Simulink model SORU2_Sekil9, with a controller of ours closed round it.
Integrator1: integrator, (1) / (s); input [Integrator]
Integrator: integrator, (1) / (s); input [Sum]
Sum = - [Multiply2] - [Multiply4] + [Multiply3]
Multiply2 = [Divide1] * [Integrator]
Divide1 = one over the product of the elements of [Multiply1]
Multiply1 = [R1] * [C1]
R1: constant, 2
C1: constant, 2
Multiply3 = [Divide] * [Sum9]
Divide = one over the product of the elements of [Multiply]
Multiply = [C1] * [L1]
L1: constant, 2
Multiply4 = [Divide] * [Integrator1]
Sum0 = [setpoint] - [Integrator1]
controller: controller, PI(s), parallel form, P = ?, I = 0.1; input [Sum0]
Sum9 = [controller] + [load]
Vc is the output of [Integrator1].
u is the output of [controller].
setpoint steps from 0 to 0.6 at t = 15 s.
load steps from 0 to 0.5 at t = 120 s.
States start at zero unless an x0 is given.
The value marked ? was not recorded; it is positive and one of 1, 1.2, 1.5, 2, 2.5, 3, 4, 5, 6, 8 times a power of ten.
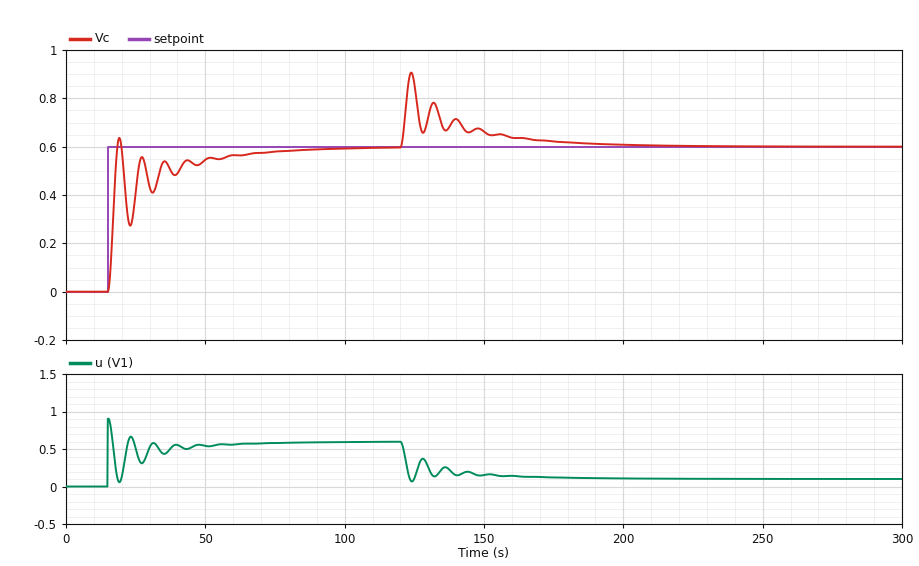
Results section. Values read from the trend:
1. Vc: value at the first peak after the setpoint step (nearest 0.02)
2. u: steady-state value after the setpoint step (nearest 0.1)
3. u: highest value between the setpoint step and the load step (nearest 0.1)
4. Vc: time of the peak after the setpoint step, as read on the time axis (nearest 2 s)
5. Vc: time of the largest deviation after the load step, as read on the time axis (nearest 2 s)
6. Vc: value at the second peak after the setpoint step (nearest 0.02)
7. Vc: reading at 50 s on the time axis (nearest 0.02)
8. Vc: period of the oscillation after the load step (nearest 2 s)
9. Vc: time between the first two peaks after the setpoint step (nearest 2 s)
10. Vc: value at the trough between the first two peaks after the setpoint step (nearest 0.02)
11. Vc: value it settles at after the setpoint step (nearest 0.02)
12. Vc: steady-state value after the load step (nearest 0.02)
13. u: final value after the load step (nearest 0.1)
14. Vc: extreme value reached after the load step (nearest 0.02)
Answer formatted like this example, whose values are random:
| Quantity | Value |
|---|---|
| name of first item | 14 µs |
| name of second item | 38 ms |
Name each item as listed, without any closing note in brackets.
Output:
| Quantity | Value |
|---|---|
| Vc: value at the first peak after the setpoint step | 0.64 |
| u: steady-state value after the setpoint step | 0.6 |
| u: highest value between the setpoint step and the load step | 0.9 |
| Vc: time of the peak after the setpoint step, as read on the time axis | 20 s |
| Vc: time of the largest deviation after the load step, as read on the time axis | 124 s |
| Vc: value at the second peak after the setpoint step | 0.56 |
| Vc: reading at 50 s on the time axis | 0.54 |
| Vc: period of the oscillation after the load step | 8 s |
| Vc: time between the first two peaks after the setpoint step | 8 s |
| Vc: value at the trough between the first two peaks after the setpoint step | 0.28 |
| Vc: value it settles at after the setpoint step | 0.60 |
| Vc: steady-state value after the load step | 0.60 |
| u: final value after the load step | 0.1 |
| Vc: extreme value reached after the load step | 0.90 |
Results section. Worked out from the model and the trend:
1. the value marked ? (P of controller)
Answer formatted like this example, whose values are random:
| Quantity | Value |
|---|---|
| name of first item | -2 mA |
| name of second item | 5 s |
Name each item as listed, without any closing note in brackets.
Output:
| Quantity | Value |
|---|---|
| the value marked ? | 1.5 |
